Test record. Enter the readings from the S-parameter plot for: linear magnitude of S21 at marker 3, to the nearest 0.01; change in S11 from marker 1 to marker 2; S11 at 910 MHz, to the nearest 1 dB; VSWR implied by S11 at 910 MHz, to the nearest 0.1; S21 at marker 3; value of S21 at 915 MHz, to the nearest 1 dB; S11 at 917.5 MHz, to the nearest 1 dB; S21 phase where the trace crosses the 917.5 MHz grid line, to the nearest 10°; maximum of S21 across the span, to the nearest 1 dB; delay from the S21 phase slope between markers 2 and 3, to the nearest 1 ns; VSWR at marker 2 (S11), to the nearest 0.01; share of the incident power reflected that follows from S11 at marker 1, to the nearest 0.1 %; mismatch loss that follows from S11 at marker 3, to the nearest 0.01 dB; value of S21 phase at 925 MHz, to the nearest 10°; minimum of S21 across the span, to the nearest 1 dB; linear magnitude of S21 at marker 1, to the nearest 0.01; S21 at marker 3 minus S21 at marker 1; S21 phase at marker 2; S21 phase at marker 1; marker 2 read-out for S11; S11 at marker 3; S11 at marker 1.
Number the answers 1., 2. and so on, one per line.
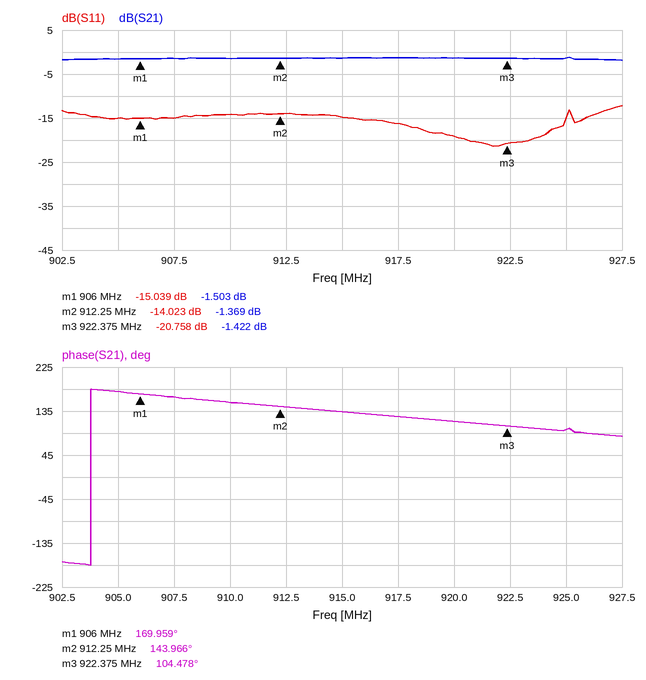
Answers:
1. 0.85
2. 1.016 dB
3. -14 dB
4. 1.5
5. -1.422 dB
6. -1 dB
7. -16 dB
8. 120°
9. -1 dB
10. 11 ns
11. 1.50
12. 3.1 %
13. 0.04 dB
14. 100°
15. -2 dB
16. 0.84
17. 0.081 dB
18. 143.966°
19. 169.959°
20. -14.023 dB
21. -20.758 dB
22. -15.039 dB
